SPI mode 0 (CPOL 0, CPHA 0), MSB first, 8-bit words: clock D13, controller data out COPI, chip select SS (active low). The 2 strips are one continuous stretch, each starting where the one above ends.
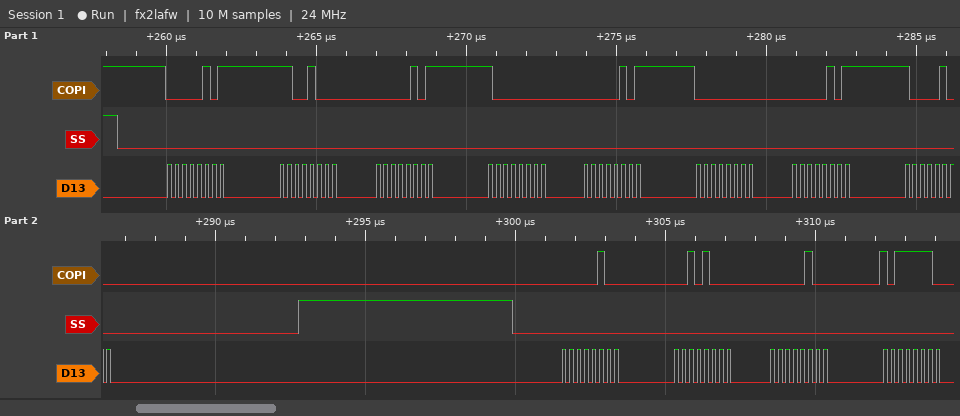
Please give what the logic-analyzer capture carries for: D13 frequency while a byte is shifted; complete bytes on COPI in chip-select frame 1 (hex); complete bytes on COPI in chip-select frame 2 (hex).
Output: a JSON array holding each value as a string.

["4 MHz", "0x05 0xC8 0x05 0x80 0x05 0x00 0x05 0x84", "0x04 0x28 0x04 0xBE"]
